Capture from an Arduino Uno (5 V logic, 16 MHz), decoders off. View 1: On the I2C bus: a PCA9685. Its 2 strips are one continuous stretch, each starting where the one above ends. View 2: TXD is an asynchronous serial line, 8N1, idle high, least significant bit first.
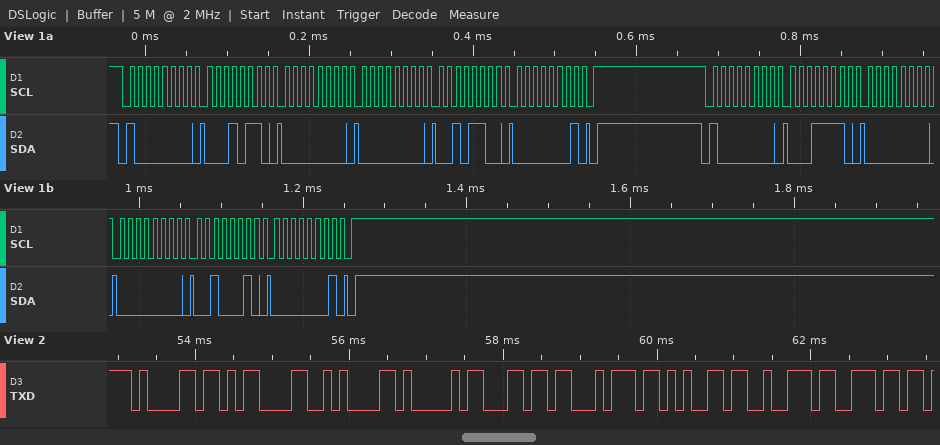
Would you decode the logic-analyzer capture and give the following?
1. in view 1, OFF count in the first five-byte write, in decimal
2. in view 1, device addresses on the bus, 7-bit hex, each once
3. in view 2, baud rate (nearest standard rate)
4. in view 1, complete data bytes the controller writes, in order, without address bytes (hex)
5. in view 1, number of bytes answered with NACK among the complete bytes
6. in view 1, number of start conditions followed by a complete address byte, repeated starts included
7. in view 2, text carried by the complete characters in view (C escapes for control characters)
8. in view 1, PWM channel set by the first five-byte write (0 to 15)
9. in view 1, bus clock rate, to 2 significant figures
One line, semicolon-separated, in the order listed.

300; 0x40; 9600 baud; 16 00 00 2C 01 1E 00 00 22 01; 0; 2; "a\r\nAltern"; 4; 100 kHz
